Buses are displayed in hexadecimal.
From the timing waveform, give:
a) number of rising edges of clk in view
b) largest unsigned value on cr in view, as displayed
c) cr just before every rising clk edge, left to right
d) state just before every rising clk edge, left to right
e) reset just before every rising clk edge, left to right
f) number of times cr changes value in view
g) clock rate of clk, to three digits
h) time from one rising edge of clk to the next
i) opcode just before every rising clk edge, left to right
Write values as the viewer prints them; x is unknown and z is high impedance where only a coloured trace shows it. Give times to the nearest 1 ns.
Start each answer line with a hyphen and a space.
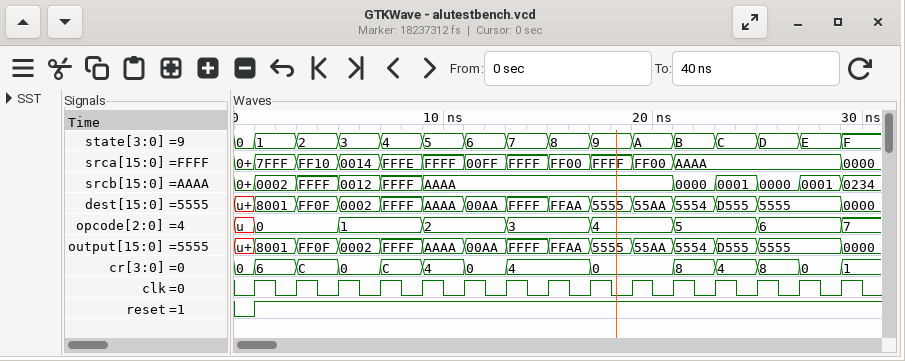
- 15
- C
- 0, 6, C, 0, C, 4, 0, 4, 4, 0, 0, 8, 4, 8, 0
- 0, 1, 2, 3, 4, 5, 6, 7, 8, 9, A, B, C, D, E
- 0 1 1 1 1 1 1 1 1 1 1 1 1 1 1
- 13
- 500 MHz
- 2 ns
- u, 0, 0, 1, 1, 2, 2, 3, 3, 4, 4, 5, 5, 6, 6
